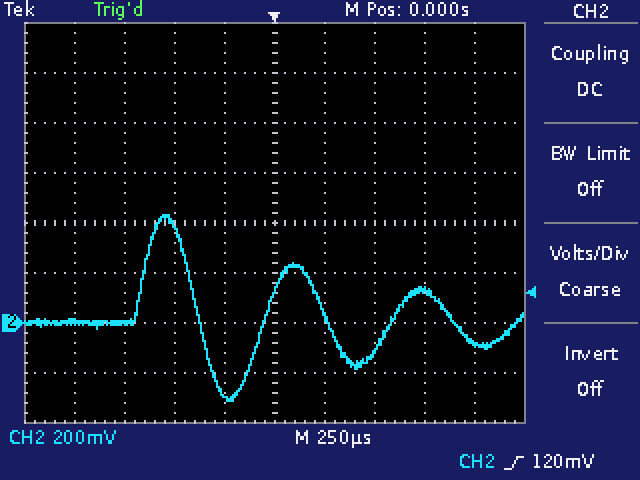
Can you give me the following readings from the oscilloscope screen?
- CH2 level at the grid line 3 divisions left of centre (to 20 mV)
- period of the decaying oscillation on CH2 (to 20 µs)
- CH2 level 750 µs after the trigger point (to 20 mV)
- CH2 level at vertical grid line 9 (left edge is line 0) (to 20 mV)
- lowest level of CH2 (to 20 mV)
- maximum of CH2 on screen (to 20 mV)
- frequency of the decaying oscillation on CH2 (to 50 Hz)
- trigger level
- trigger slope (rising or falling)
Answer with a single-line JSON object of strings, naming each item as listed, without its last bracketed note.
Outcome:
{"CH2 level at the grid line 3 divisions left of centre": "0 mV", "period of the decaying oscillation on CH2": "640 µs", "CH2 level 750 µs after the trigger point": "120 mV", "CH2 level at vertical grid line 9 (left edge is line 0)": "-80 mV", "lowest level of CH2": "-320 mV", "maximum of CH2 on screen": "440 mV", "frequency of the decaying oscillation on CH2": "1.55 kHz", "trigger level": "120 mV", "trigger slope": "rising"}
